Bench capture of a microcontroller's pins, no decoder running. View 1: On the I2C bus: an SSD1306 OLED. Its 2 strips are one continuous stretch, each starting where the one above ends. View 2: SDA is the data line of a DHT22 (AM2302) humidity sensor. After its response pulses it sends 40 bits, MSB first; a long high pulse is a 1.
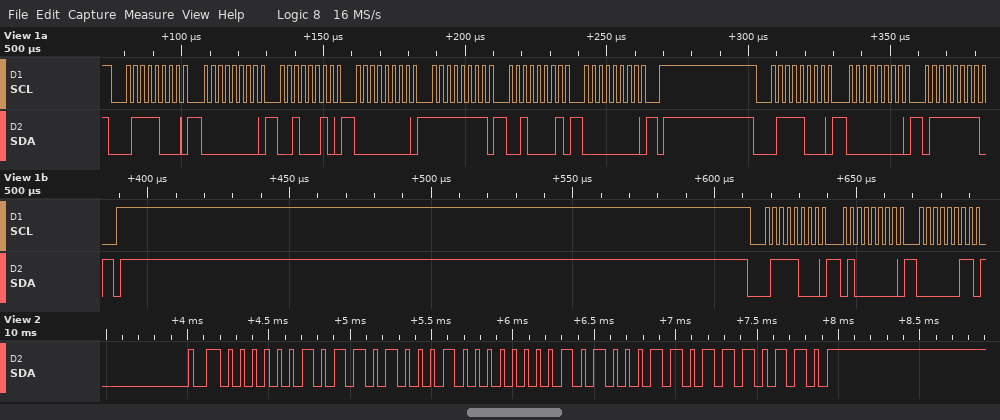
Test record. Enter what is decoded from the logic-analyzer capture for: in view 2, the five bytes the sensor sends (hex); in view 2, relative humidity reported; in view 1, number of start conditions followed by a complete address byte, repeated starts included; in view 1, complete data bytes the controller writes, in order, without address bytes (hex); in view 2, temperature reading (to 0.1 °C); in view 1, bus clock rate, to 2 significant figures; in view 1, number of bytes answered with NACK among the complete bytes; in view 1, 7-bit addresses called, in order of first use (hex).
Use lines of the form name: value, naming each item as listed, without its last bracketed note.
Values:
in view 2, the five bytes the sensor sends: 02 D1 00 A3 76
in view 2, relative humidity reported: 72.1 %
in view 1, number of start conditions followed by a complete address byte, repeated starts included: 3
in view 1, complete data bytes the controller writes, in order, without address bytes: 00 22 00 FF 21 00 00 7F 40 03
in view 2, temperature reading: 16.3 °C
in view 1, bus clock rate, to 2 significant figures: 400 kHz
in view 1, number of bytes answered with NACK among the complete bytes: 0
in view 1, 7-bit addresses called, in order of first use: 0x3C
